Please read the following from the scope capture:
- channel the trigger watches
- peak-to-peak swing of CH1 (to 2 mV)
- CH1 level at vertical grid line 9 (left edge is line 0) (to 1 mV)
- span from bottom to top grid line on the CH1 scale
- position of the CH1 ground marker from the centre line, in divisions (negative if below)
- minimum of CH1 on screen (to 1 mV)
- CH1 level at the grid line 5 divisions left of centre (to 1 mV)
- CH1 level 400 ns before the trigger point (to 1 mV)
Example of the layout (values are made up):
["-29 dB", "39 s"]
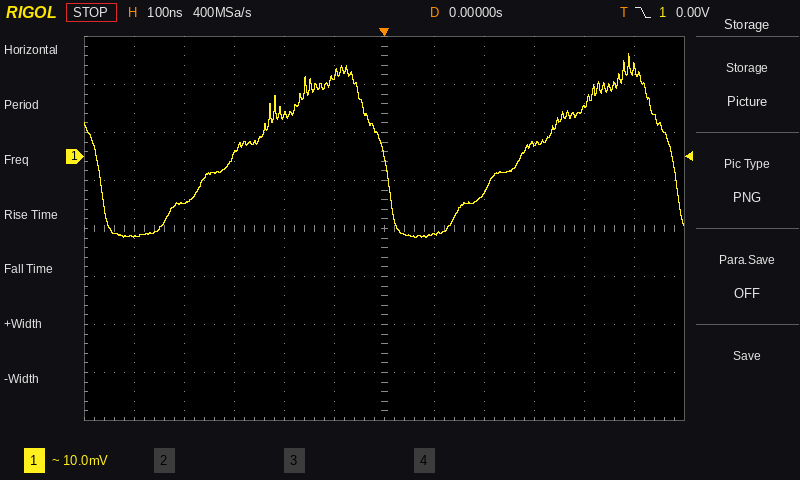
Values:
["CH1", "38 mV", "3 mV", "80 mV", "+1.5 div", "-17 mV", "-17 mV", "-10 mV"]
